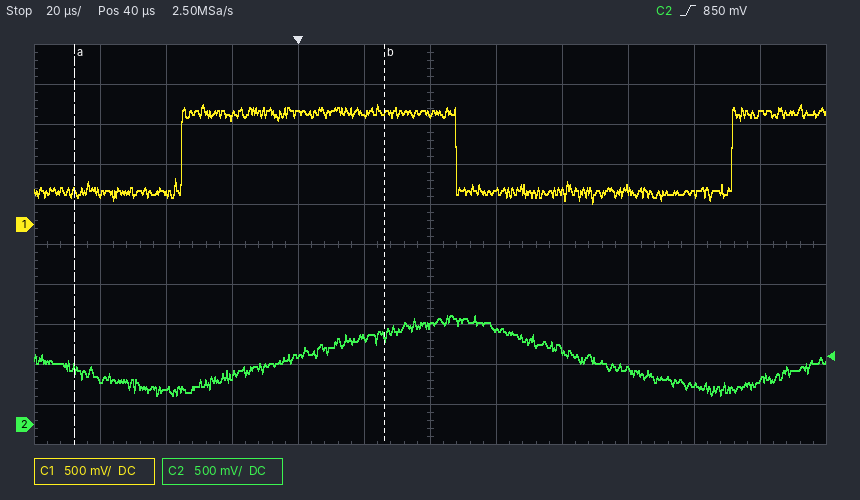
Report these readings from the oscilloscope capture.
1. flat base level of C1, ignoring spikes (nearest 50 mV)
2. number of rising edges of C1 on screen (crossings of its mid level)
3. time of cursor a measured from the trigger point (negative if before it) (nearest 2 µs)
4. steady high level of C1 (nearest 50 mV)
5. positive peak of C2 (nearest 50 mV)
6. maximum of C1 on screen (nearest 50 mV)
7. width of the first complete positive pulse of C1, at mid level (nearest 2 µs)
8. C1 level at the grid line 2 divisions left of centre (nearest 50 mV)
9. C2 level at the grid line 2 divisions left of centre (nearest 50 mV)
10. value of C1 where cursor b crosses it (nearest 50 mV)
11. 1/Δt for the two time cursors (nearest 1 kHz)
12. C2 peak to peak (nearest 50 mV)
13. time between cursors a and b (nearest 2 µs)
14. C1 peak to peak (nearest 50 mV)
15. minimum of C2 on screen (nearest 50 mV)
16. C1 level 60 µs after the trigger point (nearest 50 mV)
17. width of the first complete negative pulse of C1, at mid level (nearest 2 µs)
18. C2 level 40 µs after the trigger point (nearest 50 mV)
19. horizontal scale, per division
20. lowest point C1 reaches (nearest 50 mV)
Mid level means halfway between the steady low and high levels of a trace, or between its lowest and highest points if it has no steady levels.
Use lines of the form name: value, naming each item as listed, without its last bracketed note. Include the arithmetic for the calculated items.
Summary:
flat base level of C1, ignoring spikes: 400 mV
number of rising edges of C1 on screen: 2
time of cursor a measured from the trigger point (negative if before it): -68 µs
steady high level of C1: 1.40 V
positive peak of C2: 1.35 V
maximum of C1 on screen: 1.50 V
width of the first complete positive pulse of C1, at mid level: 84 µs
C1 level at the grid line 2 divisions left of centre: 1.40 V
C2 level at the grid line 2 divisions left of centre: 850 mV
value of C1 where cursor b crosses it: 1.40 V
1/Δt for the two time cursors: 1 / 94 µs ≈ 11 kHz
C2 peak to peak: 1.35 V − (350 mV) = 1.00 V
time between cursors a and b: 94 µs
C1 peak to peak: 1.50 V − (250 mV) = 1.25 V
minimum of C2 on screen: 350 mV
C1 level 60 µs after the trigger point: 400 mV
width of the first complete negative pulse of C1, at mid level: 84 µs
C2 level 40 µs after the trigger point: 1.25 V
horizontal scale, per division: 20 µs
lowest point C1 reaches: 250 mV
